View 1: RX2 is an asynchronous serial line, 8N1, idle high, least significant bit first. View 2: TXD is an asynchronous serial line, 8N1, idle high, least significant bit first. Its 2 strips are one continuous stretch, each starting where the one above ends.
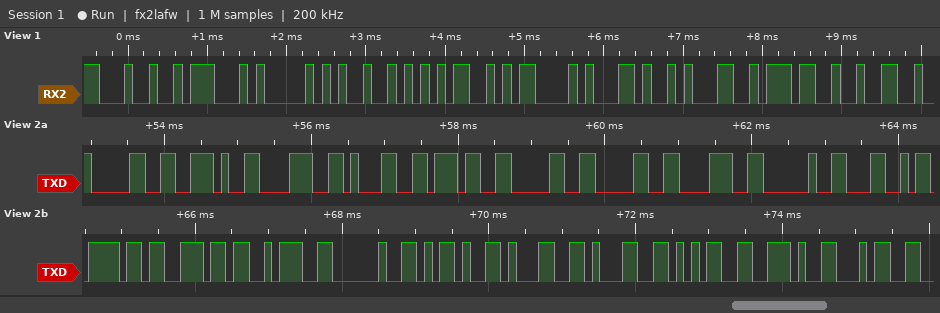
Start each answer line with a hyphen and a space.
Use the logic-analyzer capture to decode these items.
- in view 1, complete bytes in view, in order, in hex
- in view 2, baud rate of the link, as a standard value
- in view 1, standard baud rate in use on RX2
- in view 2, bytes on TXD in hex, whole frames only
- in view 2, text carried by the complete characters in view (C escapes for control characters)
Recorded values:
- 24 47 50 52 4D 43 2C 31 37 32
- 9600 baud
- 9600 baud
- 0x30 0x2E 0x38 0x31 0x37 0x30 0x30 0x38 0x20 0x4C 0x6F 0x6E 0x3A 0x20 0x2D 0x31 0x31 0x35 0x2E 0x34
- "0.817008 Lon: -115.4"
